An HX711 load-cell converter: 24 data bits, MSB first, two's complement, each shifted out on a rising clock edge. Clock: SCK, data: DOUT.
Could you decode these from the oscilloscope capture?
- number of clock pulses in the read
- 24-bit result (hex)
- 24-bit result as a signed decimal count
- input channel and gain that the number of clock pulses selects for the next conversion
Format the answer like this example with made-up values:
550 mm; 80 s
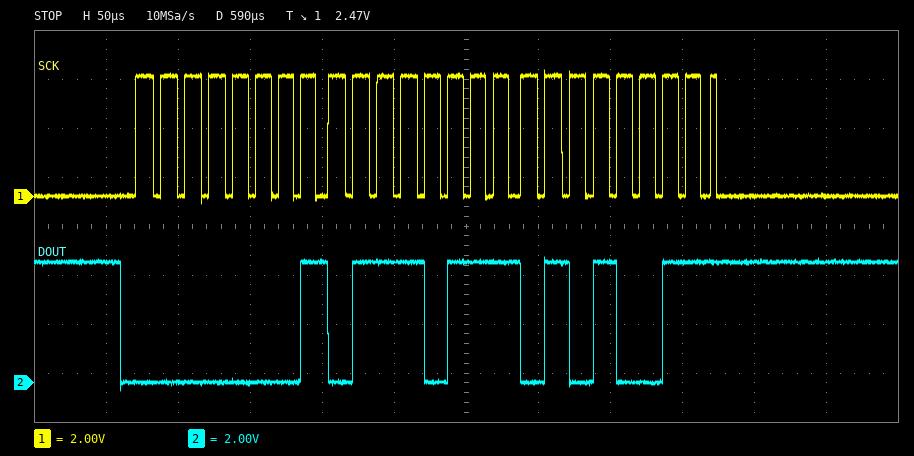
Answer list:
25; 0x017753; 96083; channel A, gain 128
